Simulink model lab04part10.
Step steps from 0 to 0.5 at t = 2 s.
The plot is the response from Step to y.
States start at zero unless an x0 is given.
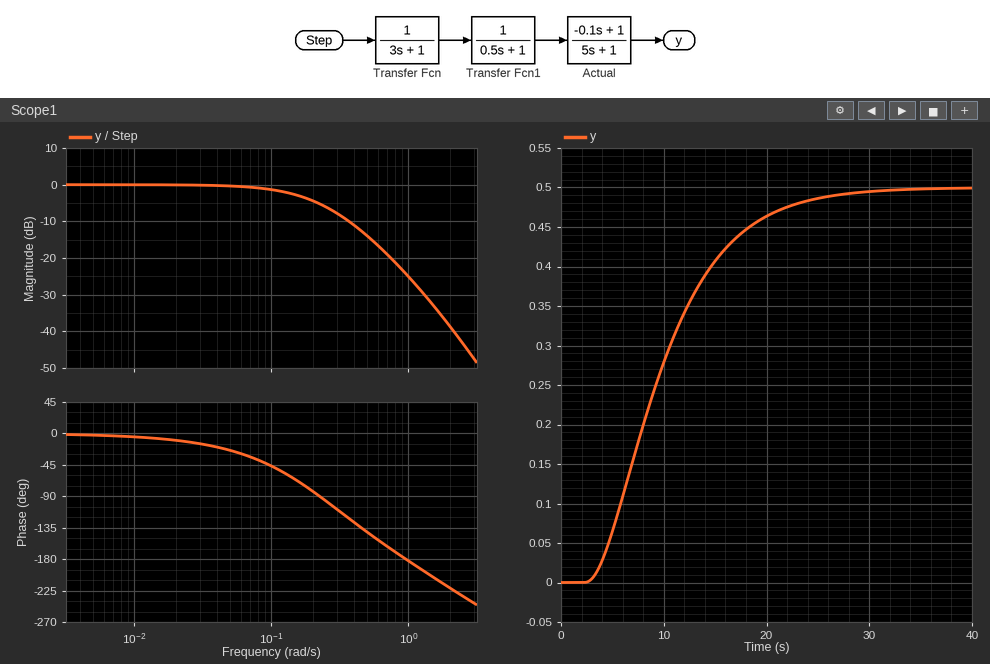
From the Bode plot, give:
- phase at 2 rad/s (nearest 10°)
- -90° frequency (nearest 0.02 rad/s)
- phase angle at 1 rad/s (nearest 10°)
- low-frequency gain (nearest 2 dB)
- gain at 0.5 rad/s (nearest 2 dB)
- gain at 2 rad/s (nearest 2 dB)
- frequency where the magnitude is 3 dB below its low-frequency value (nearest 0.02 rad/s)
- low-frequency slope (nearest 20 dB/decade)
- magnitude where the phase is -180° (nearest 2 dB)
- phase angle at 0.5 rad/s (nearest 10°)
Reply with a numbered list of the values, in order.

1. -220°
2. 0.22 rad/s
3. -180°
4. 0 dB
5. -14 dB
6. -38 dB
7. 0.16 rad/s
8. 0 dB/decade
9. -24 dB
10. -140°
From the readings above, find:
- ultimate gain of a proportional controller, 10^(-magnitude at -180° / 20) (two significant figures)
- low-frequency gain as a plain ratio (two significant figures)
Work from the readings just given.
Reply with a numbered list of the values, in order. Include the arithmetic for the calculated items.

1. 10^(24 / 20) = 16
2. 10^(0 / 20) = 1.0
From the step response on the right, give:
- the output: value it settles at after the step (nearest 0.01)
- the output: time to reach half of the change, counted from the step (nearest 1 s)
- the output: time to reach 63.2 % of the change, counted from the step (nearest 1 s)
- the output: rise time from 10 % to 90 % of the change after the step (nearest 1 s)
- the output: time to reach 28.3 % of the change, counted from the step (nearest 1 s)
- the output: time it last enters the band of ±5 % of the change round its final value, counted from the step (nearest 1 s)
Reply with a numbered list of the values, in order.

1. 0.50
2. 7 s
3. 9 s
4. 14 s
5. 5 s
6. 20 s
